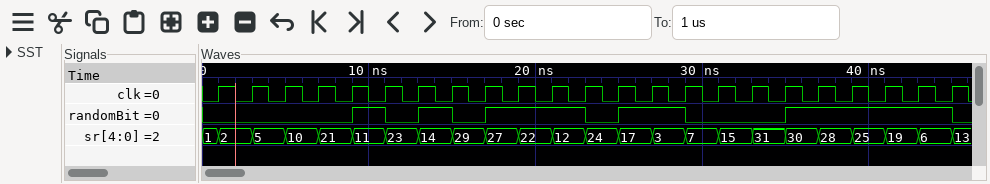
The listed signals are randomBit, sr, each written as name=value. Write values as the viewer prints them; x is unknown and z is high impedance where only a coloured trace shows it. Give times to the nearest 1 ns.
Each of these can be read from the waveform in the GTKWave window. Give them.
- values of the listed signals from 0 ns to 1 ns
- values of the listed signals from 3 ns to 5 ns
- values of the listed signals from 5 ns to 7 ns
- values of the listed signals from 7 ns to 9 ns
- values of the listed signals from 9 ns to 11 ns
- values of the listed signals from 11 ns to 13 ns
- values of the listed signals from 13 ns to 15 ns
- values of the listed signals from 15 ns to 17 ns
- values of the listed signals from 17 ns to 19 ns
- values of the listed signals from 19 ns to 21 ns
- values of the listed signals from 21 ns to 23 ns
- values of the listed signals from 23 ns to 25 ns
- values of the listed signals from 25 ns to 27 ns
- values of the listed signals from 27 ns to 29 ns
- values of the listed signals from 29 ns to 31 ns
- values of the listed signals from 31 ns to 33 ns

randomBit=0, sr=1
randomBit=0, sr=5
randomBit=0, sr=10
randomBit=0, sr=21
randomBit=1, sr=11
randomBit=0, sr=23
randomBit=1, sr=14
randomBit=0, sr=29
randomBit=1, sr=27
randomBit=1, sr=22
randomBit=1, sr=12
randomBit=0, sr=24
randomBit=1, sr=17
randomBit=1, sr=3
randomBit=0, sr=7
randomBit=0, sr=15
